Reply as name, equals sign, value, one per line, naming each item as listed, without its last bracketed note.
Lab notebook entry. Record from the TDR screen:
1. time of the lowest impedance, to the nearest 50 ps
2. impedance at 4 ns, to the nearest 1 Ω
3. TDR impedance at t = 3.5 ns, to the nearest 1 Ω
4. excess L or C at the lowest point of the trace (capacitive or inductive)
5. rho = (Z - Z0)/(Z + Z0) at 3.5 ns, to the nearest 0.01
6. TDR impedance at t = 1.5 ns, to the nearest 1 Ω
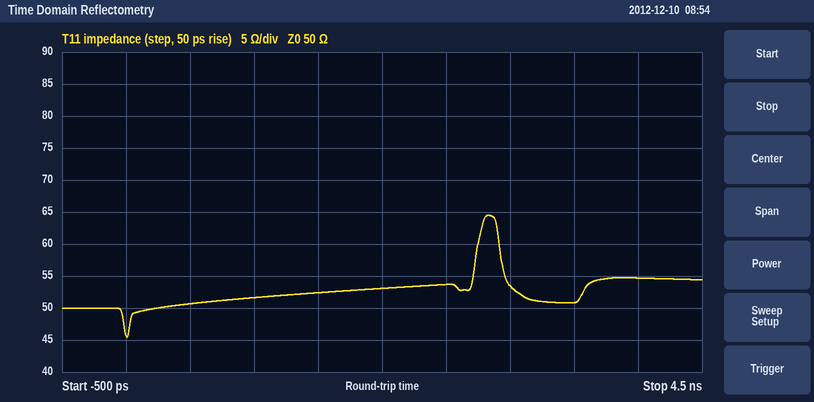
time of the lowest impedance, to the nearest 50 ps = 0 ps
impedance at 4 ns, to the nearest 1 Ω = 55 Ω
TDR impedance at t = 3.5 ns, to the nearest 1 Ω = 51 Ω
excess L or C at the lowest point of the trace = capacitive
rho = (Z - Z0)/(Z + Z0) at 3.5 ns, to the nearest 0.01 = +0.01
TDR impedance at t = 1.5 ns, to the nearest 1 Ω = 52 Ω
